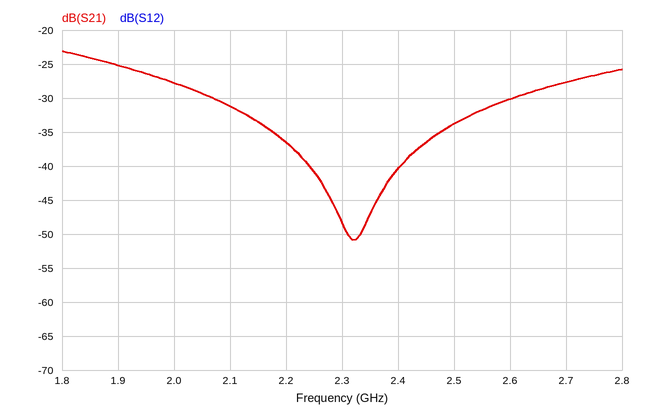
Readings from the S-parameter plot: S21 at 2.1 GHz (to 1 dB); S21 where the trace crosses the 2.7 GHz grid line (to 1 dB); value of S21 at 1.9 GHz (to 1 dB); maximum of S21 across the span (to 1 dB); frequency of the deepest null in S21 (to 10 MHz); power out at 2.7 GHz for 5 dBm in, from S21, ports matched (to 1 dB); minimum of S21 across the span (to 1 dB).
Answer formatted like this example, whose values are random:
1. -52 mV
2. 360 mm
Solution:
1. -31 dB
2. -28 dB
3. -25 dB
4. -23 dB
5. 2.32 GHz
6. -23 dBm
7. -51 dB
